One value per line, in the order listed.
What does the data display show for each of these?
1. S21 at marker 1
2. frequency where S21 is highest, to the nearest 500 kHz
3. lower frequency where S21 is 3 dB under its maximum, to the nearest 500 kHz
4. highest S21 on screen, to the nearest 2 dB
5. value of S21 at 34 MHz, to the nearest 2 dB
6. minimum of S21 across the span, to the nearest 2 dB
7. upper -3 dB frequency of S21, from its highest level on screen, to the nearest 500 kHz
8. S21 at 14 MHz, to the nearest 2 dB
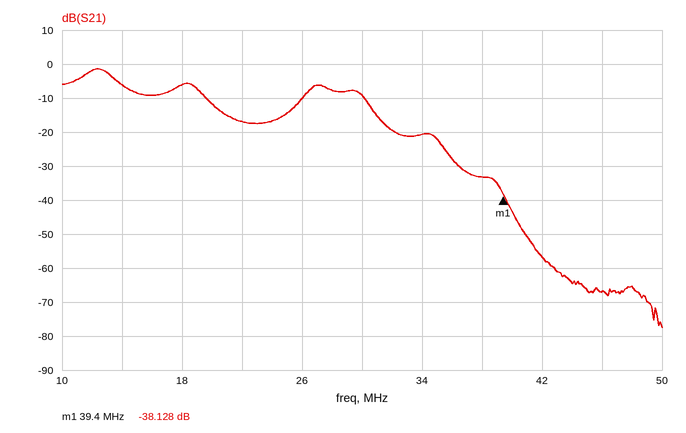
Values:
-38.128 dB
12.5 MHz
11.0 MHz
-2 dB
-20 dB
-78 dB
13.5 MHz
-6 dB
